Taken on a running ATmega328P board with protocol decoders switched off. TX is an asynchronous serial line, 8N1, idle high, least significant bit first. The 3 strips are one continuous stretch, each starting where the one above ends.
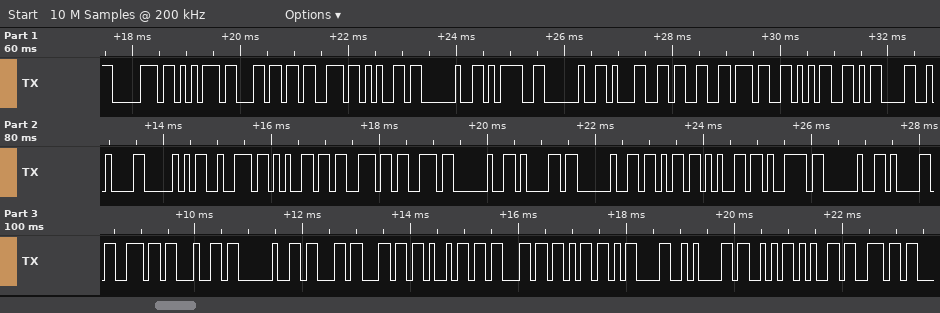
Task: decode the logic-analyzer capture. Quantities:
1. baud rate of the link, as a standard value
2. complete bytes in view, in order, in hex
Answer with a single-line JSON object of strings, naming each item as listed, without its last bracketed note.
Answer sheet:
{"baud rate of the link, as a standard value": "9600 baud", "complete bytes in view, in order, in hex": "0x70 0x75 0x6C 0x73 0x65 0x20 0x3D 0x20 0x31 0x33 0x37 0x35 0x0D 0x0A 0x50 0x72 0x65 0x73 0x73 0x20 0x61 0x20 0x6B 0x65 0x79 0x20 0x61 0x6E 0x64 0x20 0x63 0x6C 0x69 0x63 0x6B 0x0D 0x0A 0x53 0x65 0x6E"}
